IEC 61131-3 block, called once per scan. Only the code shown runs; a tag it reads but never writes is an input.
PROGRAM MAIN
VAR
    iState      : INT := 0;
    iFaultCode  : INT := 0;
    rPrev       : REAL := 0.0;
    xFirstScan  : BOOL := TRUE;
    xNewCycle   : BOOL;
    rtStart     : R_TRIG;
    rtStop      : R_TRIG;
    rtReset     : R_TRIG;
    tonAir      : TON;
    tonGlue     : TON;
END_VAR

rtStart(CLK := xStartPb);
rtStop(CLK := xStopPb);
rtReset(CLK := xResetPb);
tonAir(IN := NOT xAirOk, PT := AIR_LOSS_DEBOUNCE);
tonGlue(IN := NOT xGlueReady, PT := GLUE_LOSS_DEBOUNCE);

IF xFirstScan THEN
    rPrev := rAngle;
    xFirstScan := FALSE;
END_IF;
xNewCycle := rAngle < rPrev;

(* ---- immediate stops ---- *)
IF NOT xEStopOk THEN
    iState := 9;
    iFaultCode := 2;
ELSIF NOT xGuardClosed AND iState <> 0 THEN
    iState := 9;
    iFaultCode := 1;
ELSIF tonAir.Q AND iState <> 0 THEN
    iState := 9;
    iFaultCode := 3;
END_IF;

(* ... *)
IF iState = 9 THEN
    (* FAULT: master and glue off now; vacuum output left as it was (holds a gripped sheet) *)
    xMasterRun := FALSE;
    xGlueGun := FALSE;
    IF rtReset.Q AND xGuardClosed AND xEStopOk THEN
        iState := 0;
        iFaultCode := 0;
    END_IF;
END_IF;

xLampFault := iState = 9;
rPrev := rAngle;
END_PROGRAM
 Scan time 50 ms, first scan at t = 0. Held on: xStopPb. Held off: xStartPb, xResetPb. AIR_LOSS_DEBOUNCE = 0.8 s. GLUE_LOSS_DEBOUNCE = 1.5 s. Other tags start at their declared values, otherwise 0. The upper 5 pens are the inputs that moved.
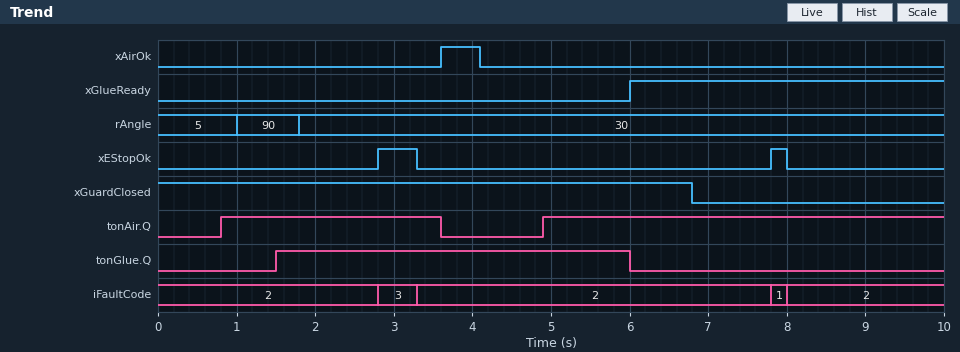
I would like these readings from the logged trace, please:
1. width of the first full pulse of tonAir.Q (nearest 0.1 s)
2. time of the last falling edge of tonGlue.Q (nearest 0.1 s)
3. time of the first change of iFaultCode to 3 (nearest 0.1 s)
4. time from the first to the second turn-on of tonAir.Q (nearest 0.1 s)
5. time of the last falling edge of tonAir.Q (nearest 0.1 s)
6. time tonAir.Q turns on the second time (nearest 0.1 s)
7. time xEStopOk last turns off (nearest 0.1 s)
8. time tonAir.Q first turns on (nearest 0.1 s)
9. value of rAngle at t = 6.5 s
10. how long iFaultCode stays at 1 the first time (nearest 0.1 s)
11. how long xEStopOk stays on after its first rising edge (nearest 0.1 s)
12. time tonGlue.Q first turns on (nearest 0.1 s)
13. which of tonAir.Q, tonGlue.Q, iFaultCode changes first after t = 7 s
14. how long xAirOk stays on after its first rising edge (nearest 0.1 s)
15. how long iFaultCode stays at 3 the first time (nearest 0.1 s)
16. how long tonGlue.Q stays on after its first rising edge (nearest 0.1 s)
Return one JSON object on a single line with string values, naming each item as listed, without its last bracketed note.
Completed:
{"width of the first full pulse of tonAir.Q": "2.8 s", "time of the last falling edge of tonGlue.Q": "6.0 s", "time of the first change of iFaultCode to 3": "2.8 s", "time from the first to the second turn-on of tonAir.Q": "4.1 s", "time of the last falling edge of tonAir.Q": "3.6 s", "time tonAir.Q turns on the second time": "4.9 s", "time xEStopOk last turns off": "8.0 s", "time tonAir.Q first turns on": "0.8 s", "value of rAngle at t = 6.5 s": "30", "how long iFaultCode stays at 1 the first time": "0.2 s", "how long xEStopOk stays on after its first rising edge": "0.5 s", "time tonGlue.Q first turns on": "1.5 s", "which of tonAir.Q, tonGlue.Q, iFaultCode changes first after t = 7 s": "iFaultCode", "how long xAirOk stays on after its first rising edge": "0.5 s", "how long iFaultCode stays at 3 the first time": "0.5 s", "how long tonGlue.Q stays on after its first rising edge": "4.5 s"}
